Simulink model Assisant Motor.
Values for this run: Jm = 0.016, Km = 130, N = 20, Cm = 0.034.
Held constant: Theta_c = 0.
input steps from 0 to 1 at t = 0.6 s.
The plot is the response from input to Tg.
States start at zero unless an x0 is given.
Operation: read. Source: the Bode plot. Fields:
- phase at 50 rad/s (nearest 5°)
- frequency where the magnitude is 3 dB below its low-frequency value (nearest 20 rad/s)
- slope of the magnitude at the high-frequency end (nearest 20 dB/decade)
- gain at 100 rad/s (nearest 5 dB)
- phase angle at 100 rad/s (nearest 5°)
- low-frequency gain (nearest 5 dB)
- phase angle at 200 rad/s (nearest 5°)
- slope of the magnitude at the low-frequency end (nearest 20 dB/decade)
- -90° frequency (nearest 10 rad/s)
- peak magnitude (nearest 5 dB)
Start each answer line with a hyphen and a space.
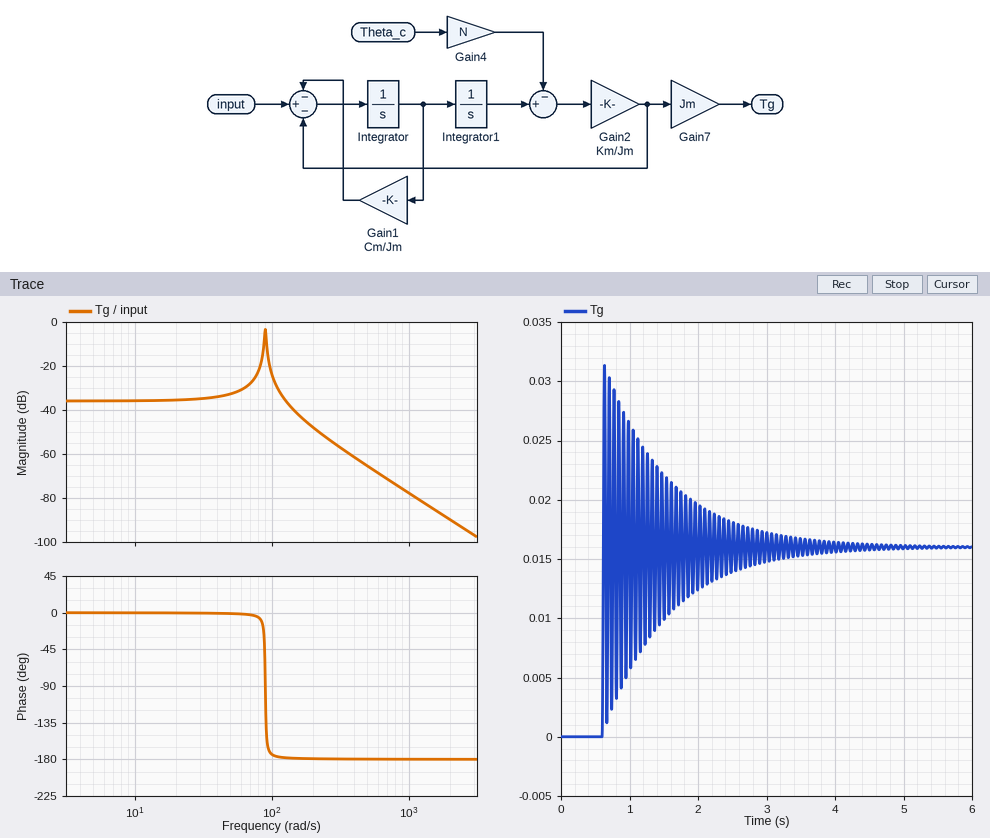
- 0°
- 140 rad/s
- -40 dB/decade
- -25 dB
- -175°
- -35 dB
- -180°
- 0 dB/decade
- 90 rad/s
- -5 dB
